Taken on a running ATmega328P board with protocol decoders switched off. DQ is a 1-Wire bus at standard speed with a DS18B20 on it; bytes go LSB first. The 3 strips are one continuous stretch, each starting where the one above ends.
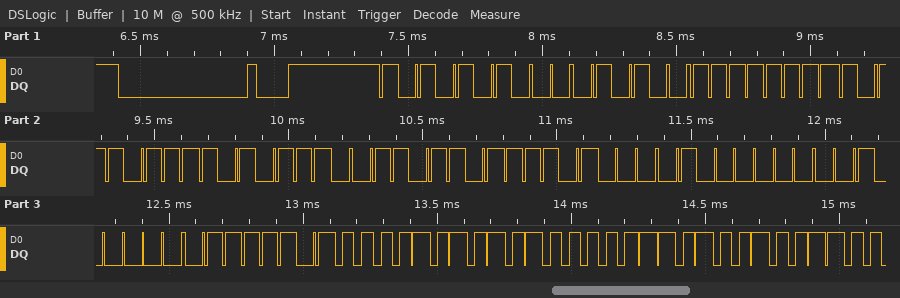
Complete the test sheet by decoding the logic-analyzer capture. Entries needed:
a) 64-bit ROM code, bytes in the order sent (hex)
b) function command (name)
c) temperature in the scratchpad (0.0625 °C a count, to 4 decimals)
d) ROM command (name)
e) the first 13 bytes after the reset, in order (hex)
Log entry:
28 FF ED 75 B6 17 02 04
Read Scratchpad
85.0000 °C
Match ROM
55 28 FF ED 75 B6 17 02 04 BE 50 05 4B
